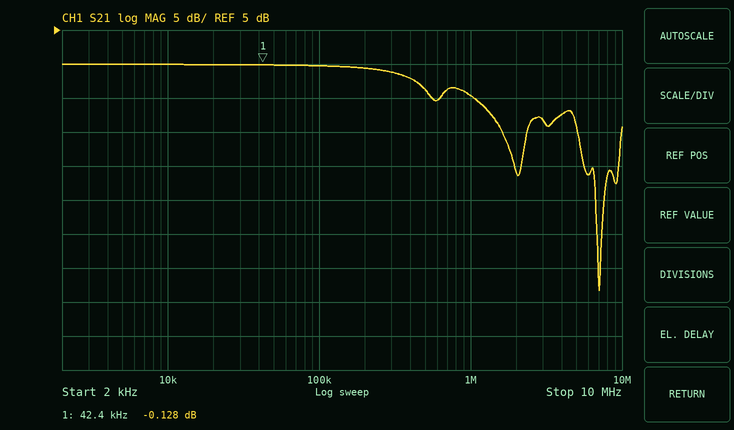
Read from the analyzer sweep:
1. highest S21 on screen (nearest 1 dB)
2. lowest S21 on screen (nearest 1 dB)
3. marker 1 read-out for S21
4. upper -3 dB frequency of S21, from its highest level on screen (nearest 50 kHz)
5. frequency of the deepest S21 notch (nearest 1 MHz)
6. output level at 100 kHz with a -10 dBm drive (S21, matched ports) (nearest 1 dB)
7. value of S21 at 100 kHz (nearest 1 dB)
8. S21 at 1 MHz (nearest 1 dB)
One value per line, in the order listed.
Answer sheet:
0 dB
-33 dB
-0.128 dB
450 kHz
7 MHz
-10 dBm
0 dB
-5 dB
